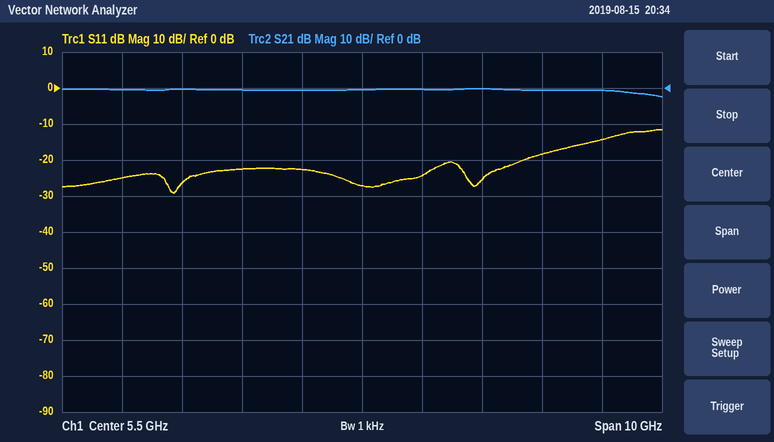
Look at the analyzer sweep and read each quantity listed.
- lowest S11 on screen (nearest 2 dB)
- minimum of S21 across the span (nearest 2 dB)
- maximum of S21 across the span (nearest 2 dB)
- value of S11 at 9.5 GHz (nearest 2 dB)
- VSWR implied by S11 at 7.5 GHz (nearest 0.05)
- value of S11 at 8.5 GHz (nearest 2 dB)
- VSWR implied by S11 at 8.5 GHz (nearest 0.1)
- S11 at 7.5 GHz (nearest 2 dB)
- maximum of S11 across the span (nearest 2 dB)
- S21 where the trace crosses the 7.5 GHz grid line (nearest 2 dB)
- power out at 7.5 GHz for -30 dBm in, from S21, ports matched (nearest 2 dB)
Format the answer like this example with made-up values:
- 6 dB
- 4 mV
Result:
- -30 dB
- -2 dB
- 0 dB
- -14 dB
- 1.10
- -18 dB
- 1.3
- -26 dB
- -12 dB
- 0 dB
- -30 dBm
